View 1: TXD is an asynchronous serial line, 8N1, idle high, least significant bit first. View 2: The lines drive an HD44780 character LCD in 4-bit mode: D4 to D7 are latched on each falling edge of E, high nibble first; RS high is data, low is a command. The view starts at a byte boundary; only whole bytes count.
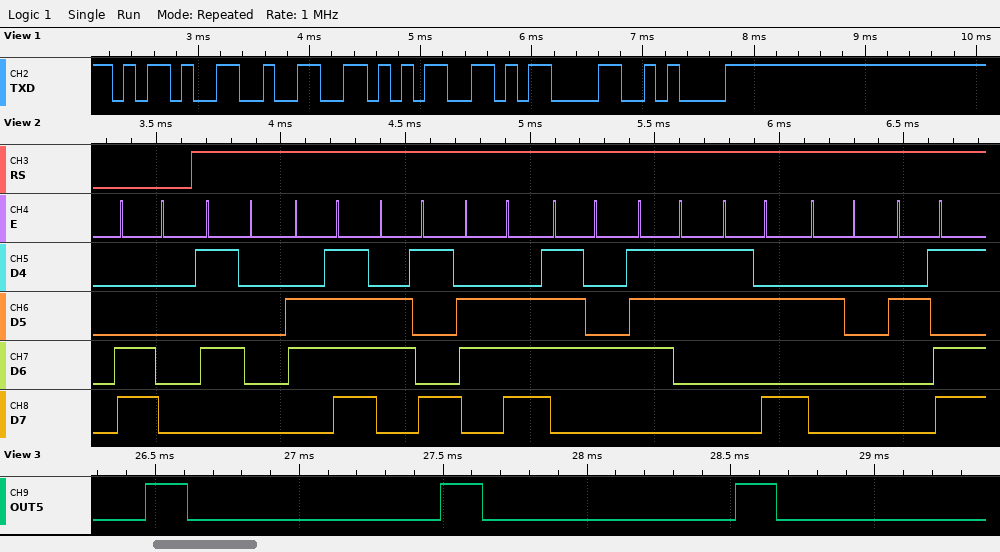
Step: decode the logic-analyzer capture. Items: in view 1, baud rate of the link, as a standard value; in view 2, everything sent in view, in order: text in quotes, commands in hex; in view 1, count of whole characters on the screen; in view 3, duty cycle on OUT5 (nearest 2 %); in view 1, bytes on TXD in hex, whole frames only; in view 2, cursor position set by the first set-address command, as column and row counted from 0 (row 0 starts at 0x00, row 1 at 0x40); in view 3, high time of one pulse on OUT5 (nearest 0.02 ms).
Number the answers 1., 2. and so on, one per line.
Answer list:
1. 9600 baud
2. 0xC0 "Points: -"
3. 5
4. 14 %
5. 2D 32 35 0D 0A
6. column 0, row 1
7. 0.14 ms
